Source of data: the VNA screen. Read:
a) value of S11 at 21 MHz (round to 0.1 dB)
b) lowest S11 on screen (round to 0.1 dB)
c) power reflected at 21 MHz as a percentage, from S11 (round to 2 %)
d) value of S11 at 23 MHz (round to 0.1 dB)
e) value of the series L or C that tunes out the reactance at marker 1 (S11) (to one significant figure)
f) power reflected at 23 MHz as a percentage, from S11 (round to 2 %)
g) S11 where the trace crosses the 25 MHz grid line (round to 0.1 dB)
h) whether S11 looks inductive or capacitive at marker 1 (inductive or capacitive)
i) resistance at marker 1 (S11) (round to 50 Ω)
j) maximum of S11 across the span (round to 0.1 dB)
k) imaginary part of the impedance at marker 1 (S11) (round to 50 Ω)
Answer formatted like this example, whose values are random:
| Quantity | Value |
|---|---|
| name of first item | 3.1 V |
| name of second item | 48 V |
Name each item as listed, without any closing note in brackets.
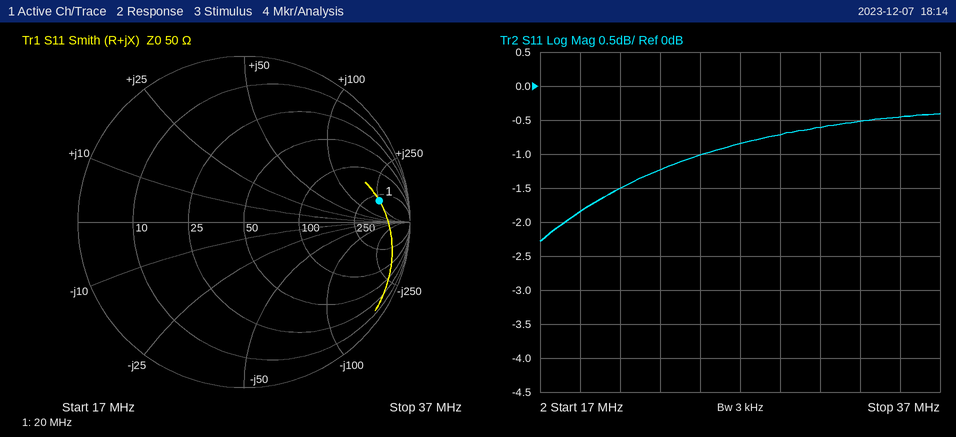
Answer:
| Quantity | Value |
|---|---|
| value of S11 at 21 MHz | -1.5 dB |
| lowest S11 on screen | -2.3 dB |
| power reflected at 21 MHz as a percentage, from S11 | 70 % |
| value of S11 at 23 MHz | -1.2 dB |
| value of the series L or C that tunes out the reactance at marker 1 (S11) | 30 pF |
| power reflected at 23 MHz as a percentage, from S11 | 76 % |
| S11 where the trace crosses the 25 MHz grid line | -1.0 dB |
| whether S11 looks inductive or capacitive at marker 1 | inductive |
| resistance at marker 1 (S11) | 300 Ω |
| maximum of S11 across the span | -0.4 dB |
| imaginary part of the impedance at marker 1 (S11) | +250 Ω |
